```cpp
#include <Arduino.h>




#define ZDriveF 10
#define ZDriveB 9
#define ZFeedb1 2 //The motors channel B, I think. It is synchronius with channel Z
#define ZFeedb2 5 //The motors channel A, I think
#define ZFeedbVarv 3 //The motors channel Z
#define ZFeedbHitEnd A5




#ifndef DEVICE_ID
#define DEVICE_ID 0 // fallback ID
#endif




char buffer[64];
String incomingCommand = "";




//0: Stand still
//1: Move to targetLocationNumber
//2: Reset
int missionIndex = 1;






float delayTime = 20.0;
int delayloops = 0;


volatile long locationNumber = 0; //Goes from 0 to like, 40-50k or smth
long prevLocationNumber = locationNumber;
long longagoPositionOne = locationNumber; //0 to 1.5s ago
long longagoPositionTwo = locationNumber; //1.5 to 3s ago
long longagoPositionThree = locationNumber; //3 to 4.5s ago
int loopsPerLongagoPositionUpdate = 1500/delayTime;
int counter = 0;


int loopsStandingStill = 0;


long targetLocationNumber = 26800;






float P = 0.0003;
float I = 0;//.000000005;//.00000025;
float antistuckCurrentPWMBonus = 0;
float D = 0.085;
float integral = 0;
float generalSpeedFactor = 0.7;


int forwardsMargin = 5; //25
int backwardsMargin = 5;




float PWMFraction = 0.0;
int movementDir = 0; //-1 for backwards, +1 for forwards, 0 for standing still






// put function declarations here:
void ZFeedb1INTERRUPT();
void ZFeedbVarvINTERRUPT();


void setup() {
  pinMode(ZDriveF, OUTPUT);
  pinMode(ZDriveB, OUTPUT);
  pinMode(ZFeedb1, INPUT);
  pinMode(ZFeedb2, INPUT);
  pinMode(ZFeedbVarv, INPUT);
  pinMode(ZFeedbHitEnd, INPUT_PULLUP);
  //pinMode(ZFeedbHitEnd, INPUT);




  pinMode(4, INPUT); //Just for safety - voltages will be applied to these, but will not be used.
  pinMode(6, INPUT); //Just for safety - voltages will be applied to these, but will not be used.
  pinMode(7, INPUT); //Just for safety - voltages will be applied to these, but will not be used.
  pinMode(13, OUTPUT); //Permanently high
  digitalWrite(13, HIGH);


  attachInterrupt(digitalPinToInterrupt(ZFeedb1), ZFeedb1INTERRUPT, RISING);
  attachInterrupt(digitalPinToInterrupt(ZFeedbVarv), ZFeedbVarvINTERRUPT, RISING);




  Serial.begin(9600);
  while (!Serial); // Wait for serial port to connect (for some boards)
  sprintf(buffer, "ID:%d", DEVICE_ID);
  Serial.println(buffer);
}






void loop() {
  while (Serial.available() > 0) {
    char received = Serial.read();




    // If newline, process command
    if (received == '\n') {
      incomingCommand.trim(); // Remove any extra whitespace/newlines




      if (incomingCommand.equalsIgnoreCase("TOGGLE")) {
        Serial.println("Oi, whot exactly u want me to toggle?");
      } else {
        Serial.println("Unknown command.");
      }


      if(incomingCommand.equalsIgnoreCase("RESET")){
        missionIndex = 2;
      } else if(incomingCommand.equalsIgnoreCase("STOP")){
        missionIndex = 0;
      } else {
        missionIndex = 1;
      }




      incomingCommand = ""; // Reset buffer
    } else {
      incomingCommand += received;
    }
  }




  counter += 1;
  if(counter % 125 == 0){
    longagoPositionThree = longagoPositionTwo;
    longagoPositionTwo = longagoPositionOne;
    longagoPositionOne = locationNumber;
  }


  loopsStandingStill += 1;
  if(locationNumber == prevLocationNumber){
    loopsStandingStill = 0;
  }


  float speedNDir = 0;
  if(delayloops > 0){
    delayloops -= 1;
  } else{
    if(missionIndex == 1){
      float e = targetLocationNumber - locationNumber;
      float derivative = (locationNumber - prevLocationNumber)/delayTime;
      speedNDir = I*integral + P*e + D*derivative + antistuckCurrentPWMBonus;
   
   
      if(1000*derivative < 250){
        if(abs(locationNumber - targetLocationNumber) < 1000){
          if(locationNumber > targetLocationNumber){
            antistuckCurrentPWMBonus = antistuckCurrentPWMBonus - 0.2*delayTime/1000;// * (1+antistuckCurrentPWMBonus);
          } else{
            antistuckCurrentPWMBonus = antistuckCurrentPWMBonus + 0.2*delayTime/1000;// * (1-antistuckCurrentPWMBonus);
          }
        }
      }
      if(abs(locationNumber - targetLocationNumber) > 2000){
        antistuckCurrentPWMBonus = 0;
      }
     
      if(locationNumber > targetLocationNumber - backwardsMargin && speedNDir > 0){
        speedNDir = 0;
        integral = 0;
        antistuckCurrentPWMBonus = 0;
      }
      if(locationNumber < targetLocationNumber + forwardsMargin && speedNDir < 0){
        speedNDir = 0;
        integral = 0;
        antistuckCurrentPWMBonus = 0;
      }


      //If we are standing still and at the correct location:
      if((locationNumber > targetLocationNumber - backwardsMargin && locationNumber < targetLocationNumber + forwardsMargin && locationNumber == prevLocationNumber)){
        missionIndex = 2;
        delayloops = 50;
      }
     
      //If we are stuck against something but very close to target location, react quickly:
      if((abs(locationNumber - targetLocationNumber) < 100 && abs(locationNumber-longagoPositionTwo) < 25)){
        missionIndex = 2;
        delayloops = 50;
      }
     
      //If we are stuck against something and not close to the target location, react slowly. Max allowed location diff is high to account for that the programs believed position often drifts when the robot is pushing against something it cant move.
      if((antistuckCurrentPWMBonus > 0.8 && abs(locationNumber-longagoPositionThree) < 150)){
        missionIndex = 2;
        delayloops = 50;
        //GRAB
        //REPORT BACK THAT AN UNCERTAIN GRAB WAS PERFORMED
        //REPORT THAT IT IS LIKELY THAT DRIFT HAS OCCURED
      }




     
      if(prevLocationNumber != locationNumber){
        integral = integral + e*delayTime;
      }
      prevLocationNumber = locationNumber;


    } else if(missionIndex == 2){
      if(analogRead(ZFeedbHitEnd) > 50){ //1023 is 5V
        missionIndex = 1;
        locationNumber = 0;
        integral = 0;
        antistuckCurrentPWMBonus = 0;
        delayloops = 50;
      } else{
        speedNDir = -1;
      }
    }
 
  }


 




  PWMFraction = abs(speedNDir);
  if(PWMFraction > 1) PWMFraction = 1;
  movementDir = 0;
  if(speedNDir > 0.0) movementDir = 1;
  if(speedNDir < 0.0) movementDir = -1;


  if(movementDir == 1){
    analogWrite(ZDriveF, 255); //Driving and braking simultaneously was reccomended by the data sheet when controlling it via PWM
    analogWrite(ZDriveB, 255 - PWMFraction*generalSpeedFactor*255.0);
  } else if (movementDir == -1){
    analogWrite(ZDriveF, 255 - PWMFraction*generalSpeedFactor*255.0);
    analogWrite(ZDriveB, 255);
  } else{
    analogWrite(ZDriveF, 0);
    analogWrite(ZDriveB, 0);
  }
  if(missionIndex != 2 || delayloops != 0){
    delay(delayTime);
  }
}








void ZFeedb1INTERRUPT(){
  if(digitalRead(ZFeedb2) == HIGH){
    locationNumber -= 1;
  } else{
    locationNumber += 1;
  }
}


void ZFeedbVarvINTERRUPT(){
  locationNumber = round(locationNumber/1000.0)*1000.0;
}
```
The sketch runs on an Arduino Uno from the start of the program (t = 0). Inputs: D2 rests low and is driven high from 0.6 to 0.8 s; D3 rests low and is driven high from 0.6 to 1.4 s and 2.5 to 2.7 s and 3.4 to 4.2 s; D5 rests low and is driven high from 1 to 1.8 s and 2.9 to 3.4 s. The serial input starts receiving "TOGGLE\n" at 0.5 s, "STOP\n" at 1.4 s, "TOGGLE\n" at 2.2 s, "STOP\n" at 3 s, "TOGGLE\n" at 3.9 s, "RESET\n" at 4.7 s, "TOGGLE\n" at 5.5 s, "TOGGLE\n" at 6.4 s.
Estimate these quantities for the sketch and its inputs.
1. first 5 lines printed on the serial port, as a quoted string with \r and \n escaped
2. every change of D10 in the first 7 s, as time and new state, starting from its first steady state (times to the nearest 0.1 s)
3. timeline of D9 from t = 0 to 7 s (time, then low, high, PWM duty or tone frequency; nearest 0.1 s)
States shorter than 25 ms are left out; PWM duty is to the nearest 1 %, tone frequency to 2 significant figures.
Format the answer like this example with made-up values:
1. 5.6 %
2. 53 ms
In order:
1. "ID:0\r\nOi, whot exactly u want me to toggle?\r\nUnknown command.\r\nOi, whot exactly u want me to toggle?\r\nUnknown command.\r\n"
2. 0 s high; 1.4 s low; 2.2 s high; 3 s low; 3.9 s high; 4.7 s PWM 30 %; 5.5 s high
3. 0 s PWM 30 %; 1.4 s low; 2.2 s PWM 30 %; 3 s low; 3.9 s PWM 30 %; 4.7 s high; 5.5 s PWM 30 %
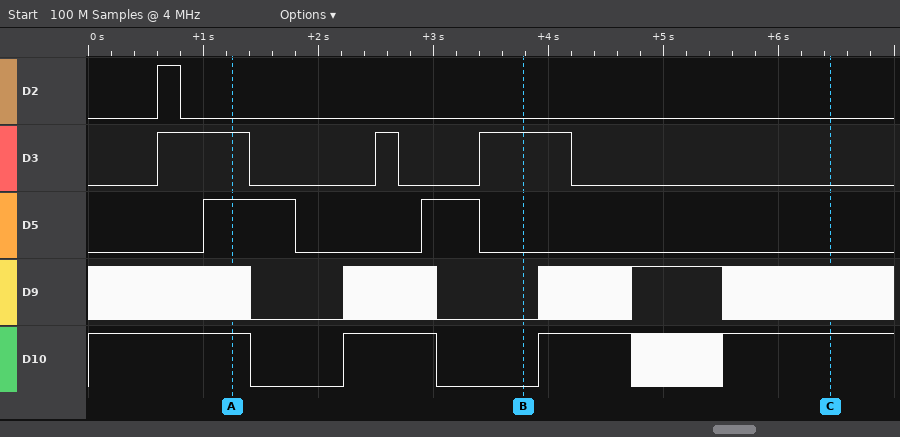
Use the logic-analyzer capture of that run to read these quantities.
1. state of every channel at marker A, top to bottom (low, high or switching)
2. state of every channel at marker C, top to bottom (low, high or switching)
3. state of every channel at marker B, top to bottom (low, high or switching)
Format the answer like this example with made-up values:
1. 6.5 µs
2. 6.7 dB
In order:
1. D2 low, D3 high, D5 high, D9 switching, D10 high
2. D2 low, D3 low, D5 low, D9 switching, D10 high
3. D2 low, D3 high, D5 low, D9 low, D10 low
